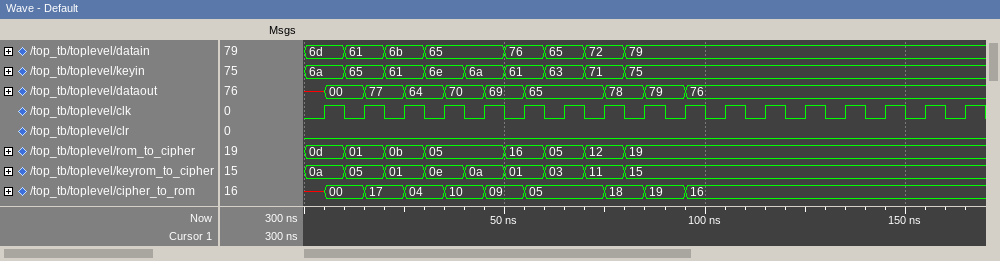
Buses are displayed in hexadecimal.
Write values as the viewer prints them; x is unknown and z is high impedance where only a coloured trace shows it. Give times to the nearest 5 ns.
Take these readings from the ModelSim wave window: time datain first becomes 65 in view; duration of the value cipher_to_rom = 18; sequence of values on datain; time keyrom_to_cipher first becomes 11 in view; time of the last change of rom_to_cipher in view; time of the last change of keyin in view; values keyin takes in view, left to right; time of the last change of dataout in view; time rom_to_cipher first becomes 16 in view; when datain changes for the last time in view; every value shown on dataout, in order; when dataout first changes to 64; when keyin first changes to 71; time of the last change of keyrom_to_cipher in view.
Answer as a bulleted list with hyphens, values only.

- 30 ns
- 10 ns
- 6d, 61, 6b, 65, 76, 65, 72, 79
- 70 ns
- 80 ns
- 80 ns
- 6a, 65, 61, 6e, 6a, 61, 63, 71, 75
- 95 ns
- 50 ns
- 80 ns
- x, 00, 77, 64, 70, 69, 65, 78, 79, 76
- 25 ns
- 70 ns
- 80 ns
